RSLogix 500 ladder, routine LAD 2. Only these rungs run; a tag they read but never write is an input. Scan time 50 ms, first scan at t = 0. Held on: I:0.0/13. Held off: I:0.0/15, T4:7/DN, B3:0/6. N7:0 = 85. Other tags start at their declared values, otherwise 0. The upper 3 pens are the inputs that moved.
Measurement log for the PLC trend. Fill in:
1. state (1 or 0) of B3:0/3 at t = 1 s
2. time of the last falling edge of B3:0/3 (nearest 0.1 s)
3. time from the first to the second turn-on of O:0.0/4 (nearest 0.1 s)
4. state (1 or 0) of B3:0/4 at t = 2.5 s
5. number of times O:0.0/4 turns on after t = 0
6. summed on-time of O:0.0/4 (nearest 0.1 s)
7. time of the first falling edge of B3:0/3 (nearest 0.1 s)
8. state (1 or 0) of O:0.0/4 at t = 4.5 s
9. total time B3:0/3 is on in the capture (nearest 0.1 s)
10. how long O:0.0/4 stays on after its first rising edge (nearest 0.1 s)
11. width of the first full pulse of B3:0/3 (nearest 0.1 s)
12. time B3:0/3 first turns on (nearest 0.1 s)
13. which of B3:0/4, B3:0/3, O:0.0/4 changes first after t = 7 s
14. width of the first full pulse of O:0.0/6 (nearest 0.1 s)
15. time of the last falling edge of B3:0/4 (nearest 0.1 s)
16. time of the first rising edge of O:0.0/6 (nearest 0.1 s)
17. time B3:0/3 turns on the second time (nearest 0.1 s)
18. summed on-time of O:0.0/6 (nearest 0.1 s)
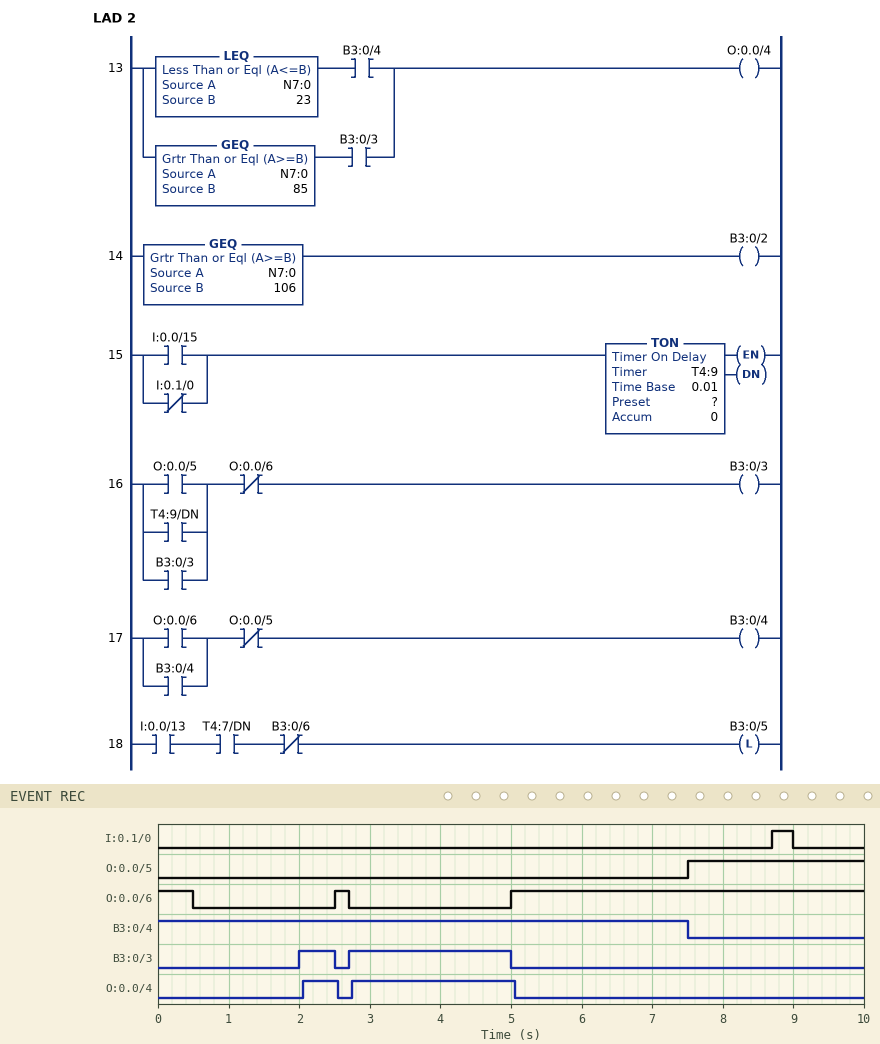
0
5.0 s
0.7 s
1
2
2.8 s
2.5 s
1
2.8 s
0.5 s
0.5 s
2.0 s
B3:0/4
0.2 s
7.5 s
2.5 s
2.7 s
5.7 s
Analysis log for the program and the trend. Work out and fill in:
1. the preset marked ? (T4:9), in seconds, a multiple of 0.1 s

2.0 s
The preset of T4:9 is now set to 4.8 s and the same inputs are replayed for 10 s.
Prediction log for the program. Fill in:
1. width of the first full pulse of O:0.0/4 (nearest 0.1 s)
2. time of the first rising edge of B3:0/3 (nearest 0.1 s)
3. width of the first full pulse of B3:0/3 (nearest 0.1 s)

0.2 s
4.8 s
0.2 s
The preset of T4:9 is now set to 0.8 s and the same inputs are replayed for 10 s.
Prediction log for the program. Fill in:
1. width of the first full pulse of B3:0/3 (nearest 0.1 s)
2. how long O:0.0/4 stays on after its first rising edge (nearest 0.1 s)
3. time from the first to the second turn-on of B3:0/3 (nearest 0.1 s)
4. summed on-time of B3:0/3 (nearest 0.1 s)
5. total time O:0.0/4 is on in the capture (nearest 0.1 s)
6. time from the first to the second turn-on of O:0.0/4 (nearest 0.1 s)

1.7 s
1.7 s
1.9 s
4.0 s
4.0 s
1.9 s
